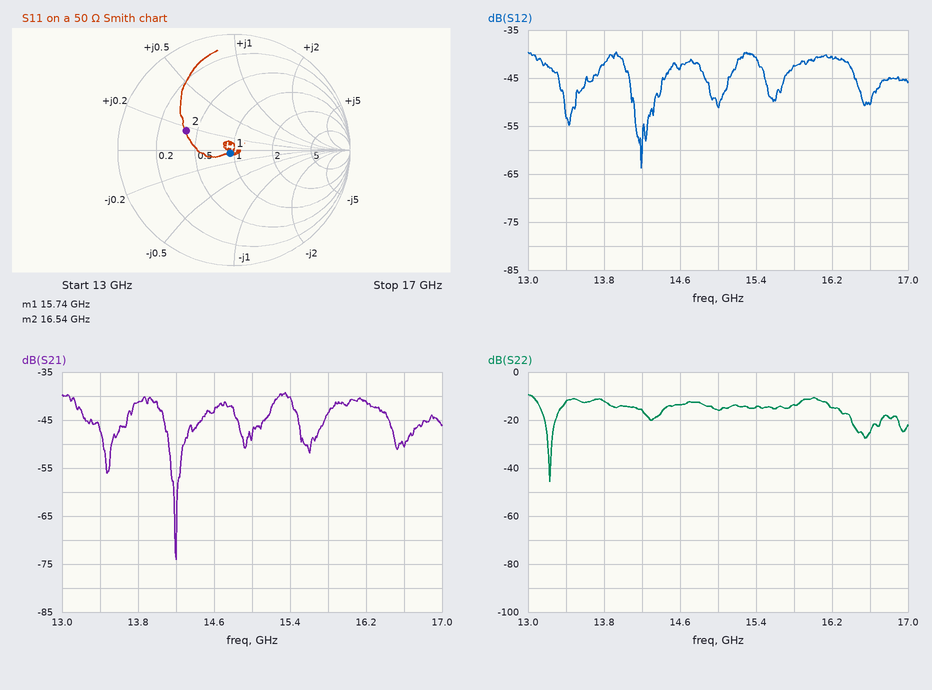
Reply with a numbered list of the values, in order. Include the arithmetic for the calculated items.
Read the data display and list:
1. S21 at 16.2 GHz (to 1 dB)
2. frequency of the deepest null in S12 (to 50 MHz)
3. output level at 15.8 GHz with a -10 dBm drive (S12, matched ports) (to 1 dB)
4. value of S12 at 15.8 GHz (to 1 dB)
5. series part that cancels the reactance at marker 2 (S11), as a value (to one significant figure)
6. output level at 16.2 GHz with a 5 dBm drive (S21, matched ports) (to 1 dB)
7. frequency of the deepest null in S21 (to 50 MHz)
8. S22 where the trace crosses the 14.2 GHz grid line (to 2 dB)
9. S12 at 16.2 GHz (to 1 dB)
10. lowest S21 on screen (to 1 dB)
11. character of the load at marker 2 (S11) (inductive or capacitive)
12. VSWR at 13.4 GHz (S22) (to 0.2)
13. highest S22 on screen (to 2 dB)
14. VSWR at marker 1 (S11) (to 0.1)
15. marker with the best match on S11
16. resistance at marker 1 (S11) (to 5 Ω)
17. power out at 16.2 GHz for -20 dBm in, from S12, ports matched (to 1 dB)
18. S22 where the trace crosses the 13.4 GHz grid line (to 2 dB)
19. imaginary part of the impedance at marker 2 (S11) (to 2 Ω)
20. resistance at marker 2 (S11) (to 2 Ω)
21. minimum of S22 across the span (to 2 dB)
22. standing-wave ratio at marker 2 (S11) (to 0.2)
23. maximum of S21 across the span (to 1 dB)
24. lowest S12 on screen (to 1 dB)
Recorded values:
1. -41 dB
2. 14.20 GHz
3. -10 dBm + (-42 dB) = -52 dBm
4. -42 dB
5. C = 1/(2π × 16.54 GHz × 8 Ω) ≈ 1 pF
6. 5 dBm + (-41 dB) = -36 dBm
7. 14.20 GHz
8. -16 dB
9. -41 dB
10. -74 dB
11. inductive
12. |Γ| = 10^(-12/20) = 0.2512; VSWR = (1 + 0.2512)/(1 − 0.2512) ≈ 1.67, so 1.6 to the nearest 0.2
13. -10 dB
14. 1.1
15. marker 1
16. 45 Ω
17. -20 dBm + (-41 dB) = -61 dBm
18. -12 dB
19. +8 Ω
20. 20 Ω
21. -46 dB
22. 2.6
23. -39 dB
24. -64 dB
